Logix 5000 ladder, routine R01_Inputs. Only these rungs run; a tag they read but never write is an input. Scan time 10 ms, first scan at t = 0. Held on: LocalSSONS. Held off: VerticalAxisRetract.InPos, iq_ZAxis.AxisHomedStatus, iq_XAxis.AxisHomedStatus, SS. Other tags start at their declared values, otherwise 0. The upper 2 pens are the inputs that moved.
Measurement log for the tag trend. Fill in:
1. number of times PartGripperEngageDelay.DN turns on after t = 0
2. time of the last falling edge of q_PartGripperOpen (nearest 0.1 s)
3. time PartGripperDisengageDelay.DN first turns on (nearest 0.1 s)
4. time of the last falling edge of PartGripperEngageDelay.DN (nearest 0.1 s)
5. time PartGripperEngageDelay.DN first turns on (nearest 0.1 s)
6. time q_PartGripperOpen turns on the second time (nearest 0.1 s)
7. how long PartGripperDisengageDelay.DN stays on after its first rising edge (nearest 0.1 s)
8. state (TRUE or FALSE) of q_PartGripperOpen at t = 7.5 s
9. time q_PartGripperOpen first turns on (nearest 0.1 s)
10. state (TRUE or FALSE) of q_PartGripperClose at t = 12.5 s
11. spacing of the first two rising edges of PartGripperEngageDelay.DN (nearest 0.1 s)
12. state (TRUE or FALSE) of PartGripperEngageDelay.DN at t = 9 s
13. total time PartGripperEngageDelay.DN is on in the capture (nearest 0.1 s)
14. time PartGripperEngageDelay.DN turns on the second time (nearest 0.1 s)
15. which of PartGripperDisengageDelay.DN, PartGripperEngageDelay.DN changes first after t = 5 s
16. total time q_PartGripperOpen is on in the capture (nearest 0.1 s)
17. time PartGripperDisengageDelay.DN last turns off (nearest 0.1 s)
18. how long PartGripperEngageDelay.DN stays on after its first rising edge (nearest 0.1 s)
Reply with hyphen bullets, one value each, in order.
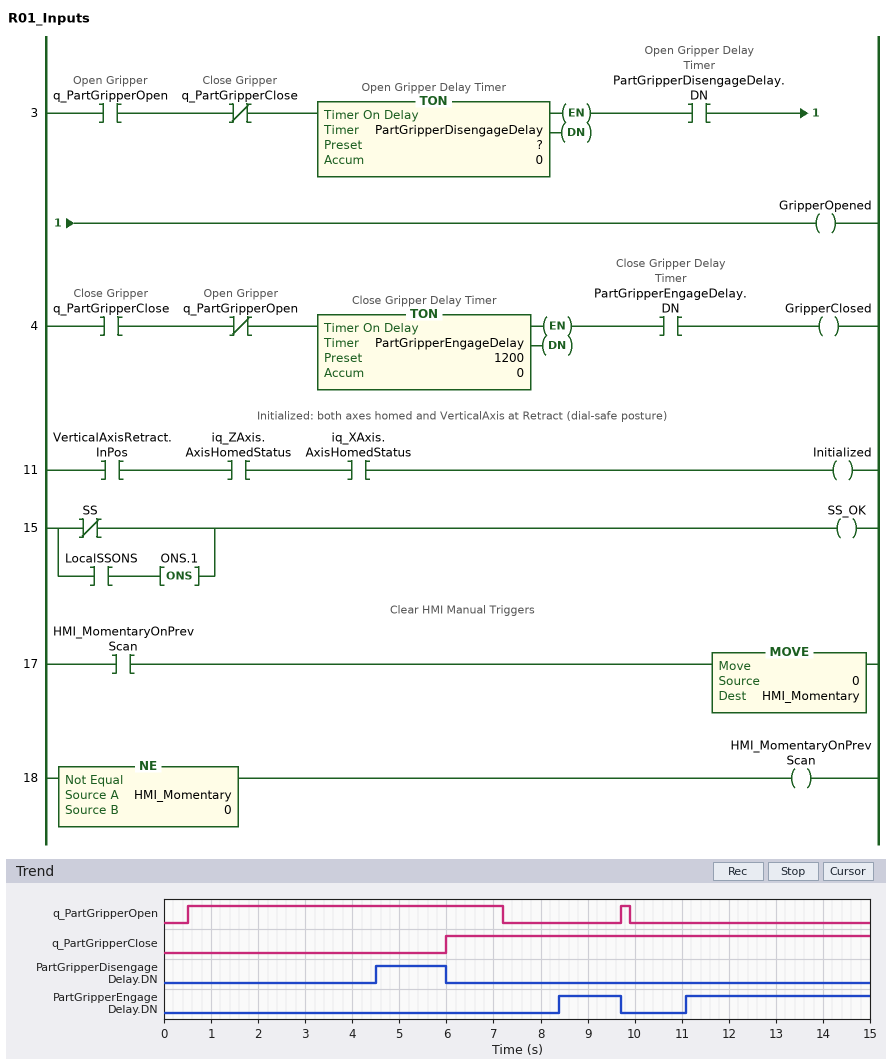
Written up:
- 2
- 9.9 s
- 4.5 s
- 9.7 s
- 8.4 s
- 9.7 s
- 1.5 s
- FALSE
- 0.5 s
- TRUE
- 2.7 s
- TRUE
- 5.2 s
- 11.1 s
- PartGripperDisengageDelay.DN
- 6.9 s
- 6.0 s
- 1.3 s
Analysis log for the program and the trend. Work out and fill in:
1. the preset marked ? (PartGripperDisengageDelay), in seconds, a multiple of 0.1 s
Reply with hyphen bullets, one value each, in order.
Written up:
- 4.0 s
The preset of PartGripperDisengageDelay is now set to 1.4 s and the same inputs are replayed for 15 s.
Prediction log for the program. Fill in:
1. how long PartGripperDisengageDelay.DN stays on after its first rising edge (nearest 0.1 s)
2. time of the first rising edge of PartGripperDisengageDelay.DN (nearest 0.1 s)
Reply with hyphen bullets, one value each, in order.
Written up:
- 4.1 s
- 1.9 s
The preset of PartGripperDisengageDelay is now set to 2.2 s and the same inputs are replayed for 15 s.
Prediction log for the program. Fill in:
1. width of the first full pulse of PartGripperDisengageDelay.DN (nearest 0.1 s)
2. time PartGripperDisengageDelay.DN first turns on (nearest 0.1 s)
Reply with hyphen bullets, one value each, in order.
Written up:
- 3.3 s
- 2.7 s
